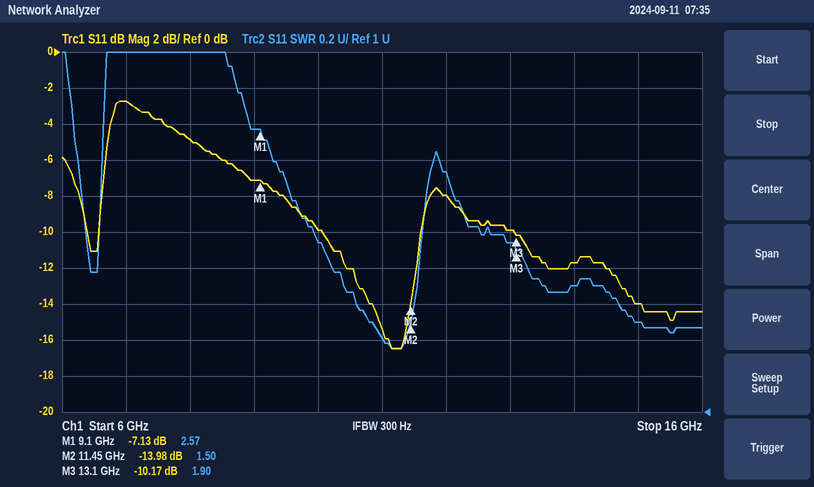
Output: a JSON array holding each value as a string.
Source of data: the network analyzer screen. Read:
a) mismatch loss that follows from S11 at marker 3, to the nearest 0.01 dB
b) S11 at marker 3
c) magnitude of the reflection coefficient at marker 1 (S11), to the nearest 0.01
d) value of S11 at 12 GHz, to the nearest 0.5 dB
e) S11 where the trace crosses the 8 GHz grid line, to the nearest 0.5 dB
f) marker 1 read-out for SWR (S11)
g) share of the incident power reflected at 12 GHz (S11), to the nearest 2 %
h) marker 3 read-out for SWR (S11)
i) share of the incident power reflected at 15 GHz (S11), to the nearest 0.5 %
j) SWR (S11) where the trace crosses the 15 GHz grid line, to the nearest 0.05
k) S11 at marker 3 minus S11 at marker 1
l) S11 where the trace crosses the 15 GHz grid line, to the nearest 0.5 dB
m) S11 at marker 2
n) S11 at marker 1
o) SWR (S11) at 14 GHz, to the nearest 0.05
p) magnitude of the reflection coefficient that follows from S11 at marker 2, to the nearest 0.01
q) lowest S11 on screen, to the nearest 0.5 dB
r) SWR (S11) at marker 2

["0.44 dB", "-10.17 dB", "0.44", "-8.0 dB", "-5.0 dB", "2.57", "16 %", "1.90", "4.0 %", "1.50", "-3.04 dB", "-14.0 dB", "-13.98 dB", "-7.13 dB", "1.70", "0.20", "-16.5 dB", "1.50"]
